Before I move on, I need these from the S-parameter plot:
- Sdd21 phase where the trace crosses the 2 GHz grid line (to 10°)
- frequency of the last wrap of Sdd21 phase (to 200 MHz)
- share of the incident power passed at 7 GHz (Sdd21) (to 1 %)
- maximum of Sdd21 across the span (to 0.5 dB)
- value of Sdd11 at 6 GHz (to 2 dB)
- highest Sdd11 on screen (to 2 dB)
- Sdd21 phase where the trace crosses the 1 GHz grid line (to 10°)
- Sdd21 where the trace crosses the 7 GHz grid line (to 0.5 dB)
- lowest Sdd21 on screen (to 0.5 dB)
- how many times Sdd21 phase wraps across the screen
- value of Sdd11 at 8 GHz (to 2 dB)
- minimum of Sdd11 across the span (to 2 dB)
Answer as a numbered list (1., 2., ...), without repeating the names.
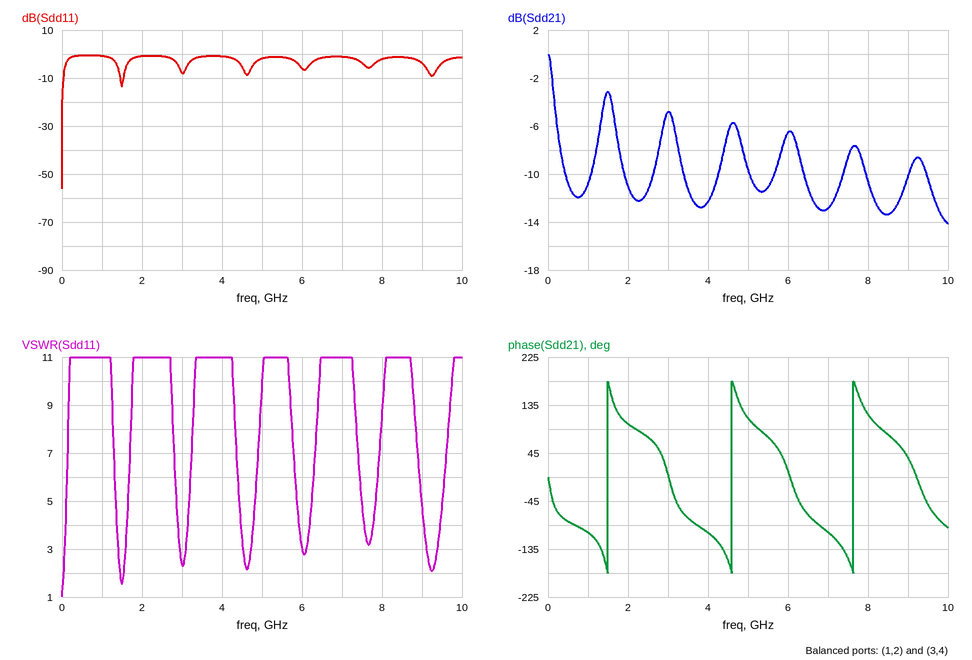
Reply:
1. 100°
2. 7.6 GHz
3. 5 %
4. 0.0 dB
5. -6 dB
6. 0 dB
7. -100°
8. -13.0 dB
9. -14.0 dB
10. 3
11. -2 dB
12. -56 dB
